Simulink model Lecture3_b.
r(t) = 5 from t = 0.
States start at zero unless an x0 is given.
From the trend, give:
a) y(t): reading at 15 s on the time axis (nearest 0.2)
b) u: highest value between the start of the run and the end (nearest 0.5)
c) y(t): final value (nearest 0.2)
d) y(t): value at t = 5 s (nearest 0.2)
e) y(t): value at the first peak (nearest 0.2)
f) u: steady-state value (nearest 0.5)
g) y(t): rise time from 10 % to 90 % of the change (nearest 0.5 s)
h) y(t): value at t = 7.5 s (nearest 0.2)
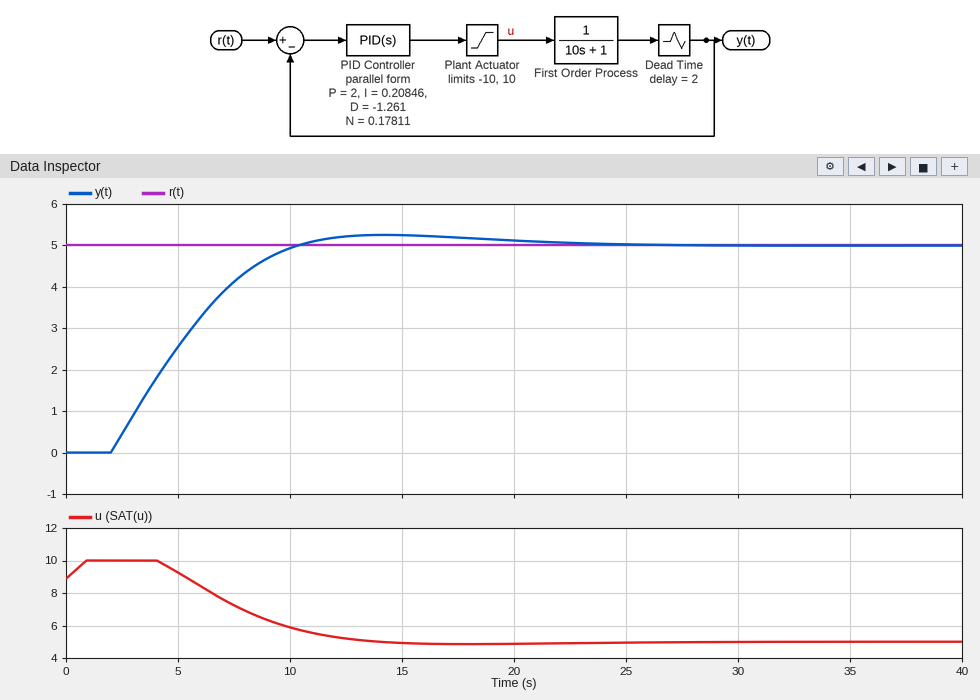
5.2
10.0
5.0
2.6
5.2
5.0
6.0 s
4.2
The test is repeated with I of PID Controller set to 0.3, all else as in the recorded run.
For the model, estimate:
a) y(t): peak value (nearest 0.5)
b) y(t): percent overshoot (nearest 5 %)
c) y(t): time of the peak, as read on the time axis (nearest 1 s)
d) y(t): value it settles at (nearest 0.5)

6.0
20 %
14 s
5.0
